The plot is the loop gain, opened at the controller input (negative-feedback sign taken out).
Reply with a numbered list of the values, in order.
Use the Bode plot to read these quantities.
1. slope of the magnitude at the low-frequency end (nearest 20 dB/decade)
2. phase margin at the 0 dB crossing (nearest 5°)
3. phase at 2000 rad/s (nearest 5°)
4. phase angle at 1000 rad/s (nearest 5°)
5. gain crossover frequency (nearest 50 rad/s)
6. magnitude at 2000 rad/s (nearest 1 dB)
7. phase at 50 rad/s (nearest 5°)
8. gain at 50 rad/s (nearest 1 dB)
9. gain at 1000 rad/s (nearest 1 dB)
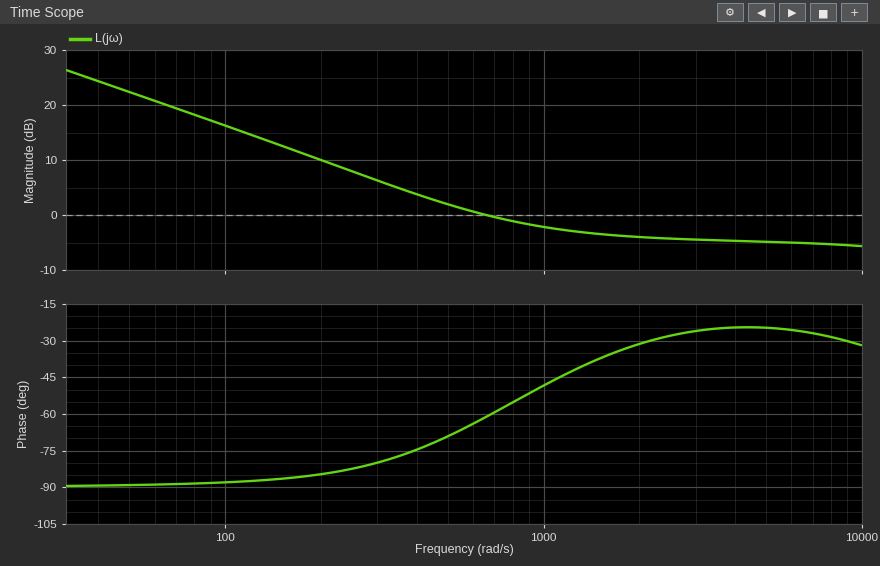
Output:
1. -20 dB/decade
2. 120°
3. -30°
4. -50°
5. 650 rad/s
6. -4 dB
7. -90°
8. 22 dB
9. -2 dB
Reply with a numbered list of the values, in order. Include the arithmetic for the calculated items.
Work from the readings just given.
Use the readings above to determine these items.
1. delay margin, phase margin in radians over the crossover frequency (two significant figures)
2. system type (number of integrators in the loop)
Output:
1. 120 × π / 180 / 650 = 0.0032 s
2. 1
